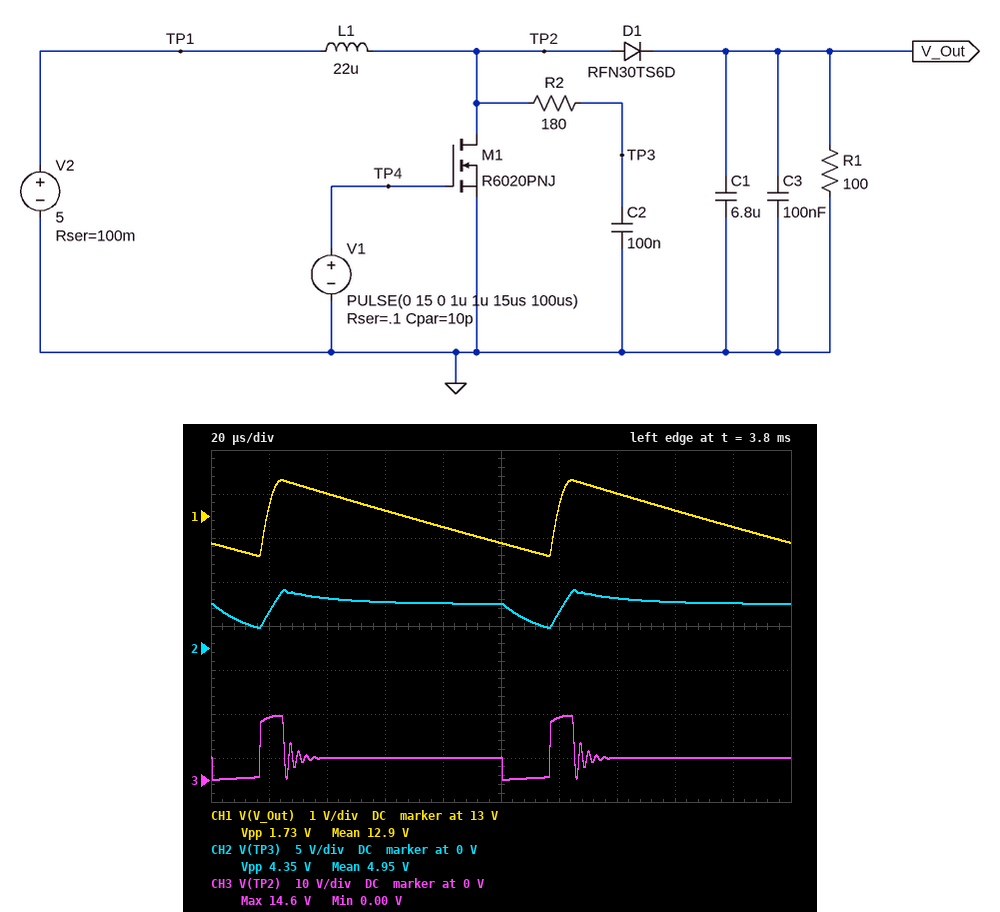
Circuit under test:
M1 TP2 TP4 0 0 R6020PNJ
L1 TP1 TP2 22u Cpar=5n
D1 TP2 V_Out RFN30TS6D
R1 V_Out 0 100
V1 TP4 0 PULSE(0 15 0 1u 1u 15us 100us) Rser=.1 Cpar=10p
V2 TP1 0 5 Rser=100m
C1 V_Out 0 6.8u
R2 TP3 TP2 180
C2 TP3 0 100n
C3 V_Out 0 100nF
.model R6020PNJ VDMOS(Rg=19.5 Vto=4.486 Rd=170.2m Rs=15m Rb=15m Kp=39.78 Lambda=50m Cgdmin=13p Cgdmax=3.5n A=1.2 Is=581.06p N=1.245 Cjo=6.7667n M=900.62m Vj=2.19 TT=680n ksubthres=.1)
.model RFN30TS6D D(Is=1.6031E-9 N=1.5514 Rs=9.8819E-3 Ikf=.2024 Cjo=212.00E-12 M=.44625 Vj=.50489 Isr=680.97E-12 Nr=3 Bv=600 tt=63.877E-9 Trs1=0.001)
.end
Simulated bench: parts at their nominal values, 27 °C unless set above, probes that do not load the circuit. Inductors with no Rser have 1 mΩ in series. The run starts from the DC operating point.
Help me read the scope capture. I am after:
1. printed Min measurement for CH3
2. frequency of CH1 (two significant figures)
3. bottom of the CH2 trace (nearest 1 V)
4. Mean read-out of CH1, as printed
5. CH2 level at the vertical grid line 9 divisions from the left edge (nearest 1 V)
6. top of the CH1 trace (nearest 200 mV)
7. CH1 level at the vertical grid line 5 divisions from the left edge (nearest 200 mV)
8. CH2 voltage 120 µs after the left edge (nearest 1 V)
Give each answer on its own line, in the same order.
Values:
0.00 V
10 kHz
2 V
12.9 V
5 V
13.8 V
12.4 V
4 V
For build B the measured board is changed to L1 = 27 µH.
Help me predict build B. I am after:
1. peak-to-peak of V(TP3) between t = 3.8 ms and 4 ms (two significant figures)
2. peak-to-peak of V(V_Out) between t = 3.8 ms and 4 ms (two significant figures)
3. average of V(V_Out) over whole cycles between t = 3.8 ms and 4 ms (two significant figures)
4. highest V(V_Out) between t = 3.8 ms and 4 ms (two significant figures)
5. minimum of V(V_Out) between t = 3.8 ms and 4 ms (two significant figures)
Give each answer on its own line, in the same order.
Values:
4.5 V
1.6 V
12 V
13 V
11 V
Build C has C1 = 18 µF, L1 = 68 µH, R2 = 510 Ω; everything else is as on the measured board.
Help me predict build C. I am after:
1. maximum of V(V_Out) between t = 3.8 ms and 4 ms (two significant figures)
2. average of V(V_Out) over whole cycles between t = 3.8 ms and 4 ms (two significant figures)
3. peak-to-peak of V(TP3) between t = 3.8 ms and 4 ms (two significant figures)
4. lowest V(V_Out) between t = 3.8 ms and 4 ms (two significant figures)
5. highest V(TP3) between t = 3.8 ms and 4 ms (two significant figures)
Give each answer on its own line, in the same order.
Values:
9.2 V
9.0 V
1.7 V
8.8 V
5.4 V
